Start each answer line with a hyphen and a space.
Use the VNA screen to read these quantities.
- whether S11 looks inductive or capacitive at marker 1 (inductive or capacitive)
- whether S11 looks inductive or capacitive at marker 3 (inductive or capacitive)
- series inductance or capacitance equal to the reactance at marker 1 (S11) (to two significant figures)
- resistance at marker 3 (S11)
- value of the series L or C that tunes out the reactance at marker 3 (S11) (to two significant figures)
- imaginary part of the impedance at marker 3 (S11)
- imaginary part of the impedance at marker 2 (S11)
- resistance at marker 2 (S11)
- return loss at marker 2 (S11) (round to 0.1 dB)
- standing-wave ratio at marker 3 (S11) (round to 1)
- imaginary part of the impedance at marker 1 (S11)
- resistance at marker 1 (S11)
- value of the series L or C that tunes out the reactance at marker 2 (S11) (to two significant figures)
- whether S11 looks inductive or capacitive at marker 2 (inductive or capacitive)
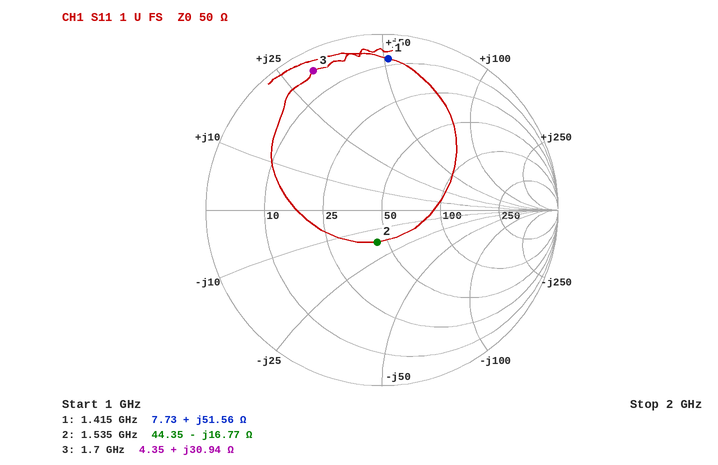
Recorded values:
- inductive
- inductive
- 5.8 nH
- 4.35 Ω
- 3.0 pF
- +30.94 Ω
- -16.77 Ω
- 44.35 Ω
- 14.7 dB
- 16
- +51.56 Ω
- 7.73 Ω
- 1.7 nH
- capacitive
